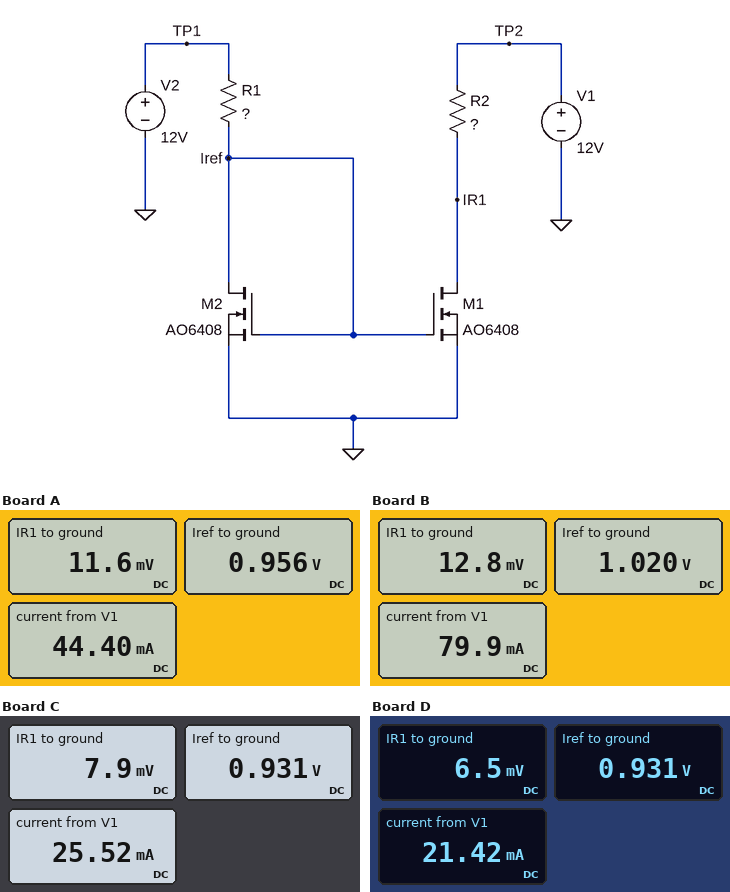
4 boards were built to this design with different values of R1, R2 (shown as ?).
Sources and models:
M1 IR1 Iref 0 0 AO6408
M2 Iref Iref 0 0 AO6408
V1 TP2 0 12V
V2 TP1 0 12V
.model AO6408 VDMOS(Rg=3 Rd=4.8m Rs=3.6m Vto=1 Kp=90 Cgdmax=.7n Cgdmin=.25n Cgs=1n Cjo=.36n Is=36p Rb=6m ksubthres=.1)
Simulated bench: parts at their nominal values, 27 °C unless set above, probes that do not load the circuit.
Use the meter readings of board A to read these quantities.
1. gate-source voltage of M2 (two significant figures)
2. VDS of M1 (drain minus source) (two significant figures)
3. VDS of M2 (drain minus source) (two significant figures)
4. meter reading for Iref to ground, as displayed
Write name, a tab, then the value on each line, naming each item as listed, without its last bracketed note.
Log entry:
gate-source voltage of M2	960 mV
VDS of M1 (drain minus source)	12 mV
VDS of M2 (drain minus source)	960 mV
meter reading for Iref to ground, as displayed	0.956 V
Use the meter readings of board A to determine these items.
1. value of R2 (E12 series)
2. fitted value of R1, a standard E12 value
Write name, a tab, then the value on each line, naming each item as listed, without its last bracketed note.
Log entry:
value of R2	270 Ω
fitted value of R1, a standard E12 value	100 Ω
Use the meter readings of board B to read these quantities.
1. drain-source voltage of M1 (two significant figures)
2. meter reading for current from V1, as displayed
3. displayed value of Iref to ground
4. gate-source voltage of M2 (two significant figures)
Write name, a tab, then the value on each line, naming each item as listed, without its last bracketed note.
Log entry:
drain-source voltage of M1	13 mV
meter reading for current from V1, as displayed	79.9 mA
displayed value of Iref to ground	1.020 V
gate-source voltage of M2	1.0 V
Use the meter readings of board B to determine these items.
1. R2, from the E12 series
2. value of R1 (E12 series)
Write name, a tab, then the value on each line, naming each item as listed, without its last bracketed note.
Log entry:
R2, from the E12 series	150 Ω
value of R1	39 Ω
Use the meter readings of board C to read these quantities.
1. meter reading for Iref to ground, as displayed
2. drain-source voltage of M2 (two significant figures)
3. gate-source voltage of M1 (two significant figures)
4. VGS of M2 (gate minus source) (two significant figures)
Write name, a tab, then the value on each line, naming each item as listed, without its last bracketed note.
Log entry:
meter reading for Iref to ground, as displayed	0.931 V
drain-source voltage of M2	930 mV
gate-source voltage of M1	930 mV
VGS of M2 (gate minus source)	930 mV
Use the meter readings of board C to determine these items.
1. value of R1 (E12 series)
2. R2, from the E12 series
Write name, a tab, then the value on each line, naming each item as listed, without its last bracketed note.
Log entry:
value of R1	150 Ω
R2, from the E12 series	470 Ω
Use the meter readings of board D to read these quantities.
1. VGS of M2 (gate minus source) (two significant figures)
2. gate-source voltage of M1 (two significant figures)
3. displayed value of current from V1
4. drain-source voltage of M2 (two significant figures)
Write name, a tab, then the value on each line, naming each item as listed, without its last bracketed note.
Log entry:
VGS of M2 (gate minus source)	930 mV
gate-source voltage of M1	930 mV
displayed value of current from V1	21.42 mA
drain-source voltage of M2	930 mV
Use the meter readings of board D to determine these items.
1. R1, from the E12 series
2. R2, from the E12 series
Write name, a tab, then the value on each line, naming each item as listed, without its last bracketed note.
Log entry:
R1, from the E12 series	150 Ω
R2, from the E12 series	560 Ω
